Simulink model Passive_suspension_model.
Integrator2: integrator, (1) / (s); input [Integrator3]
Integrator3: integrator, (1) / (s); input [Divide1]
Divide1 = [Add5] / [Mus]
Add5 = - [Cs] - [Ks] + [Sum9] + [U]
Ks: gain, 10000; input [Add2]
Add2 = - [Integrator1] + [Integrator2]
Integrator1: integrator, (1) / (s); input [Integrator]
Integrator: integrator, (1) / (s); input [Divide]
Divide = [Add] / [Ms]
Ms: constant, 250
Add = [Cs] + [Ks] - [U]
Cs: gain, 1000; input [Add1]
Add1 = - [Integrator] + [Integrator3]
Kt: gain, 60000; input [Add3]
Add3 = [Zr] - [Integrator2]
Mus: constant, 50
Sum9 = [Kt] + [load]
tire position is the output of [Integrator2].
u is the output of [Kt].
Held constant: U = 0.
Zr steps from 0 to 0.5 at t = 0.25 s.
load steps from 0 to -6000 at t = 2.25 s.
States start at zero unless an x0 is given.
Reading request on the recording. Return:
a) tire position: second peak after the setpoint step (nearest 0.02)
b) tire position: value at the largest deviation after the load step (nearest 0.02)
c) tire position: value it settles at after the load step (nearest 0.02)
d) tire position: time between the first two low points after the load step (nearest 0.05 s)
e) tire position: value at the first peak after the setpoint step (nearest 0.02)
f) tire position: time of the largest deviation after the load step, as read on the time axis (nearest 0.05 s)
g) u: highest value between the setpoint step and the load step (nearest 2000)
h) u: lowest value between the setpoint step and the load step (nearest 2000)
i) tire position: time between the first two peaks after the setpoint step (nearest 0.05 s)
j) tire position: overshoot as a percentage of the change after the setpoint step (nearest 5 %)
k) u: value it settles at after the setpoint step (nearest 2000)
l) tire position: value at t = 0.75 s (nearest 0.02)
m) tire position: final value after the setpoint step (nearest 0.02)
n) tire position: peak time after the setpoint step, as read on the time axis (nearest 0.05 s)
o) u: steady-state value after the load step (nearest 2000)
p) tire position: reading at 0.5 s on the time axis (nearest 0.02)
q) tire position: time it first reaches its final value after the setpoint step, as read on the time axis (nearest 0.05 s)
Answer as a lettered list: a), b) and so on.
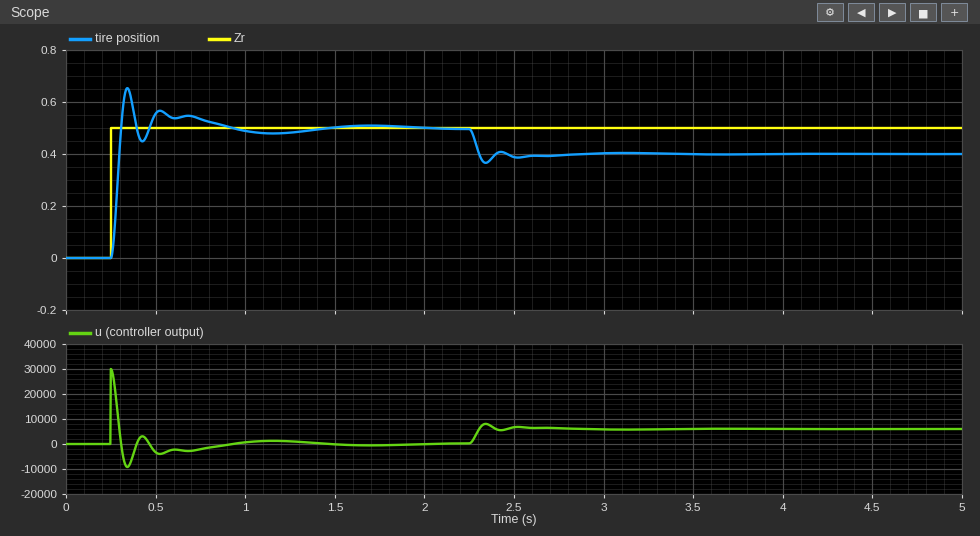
a) 0.56
b) 0.36
c) 0.40
d) 0.20 s
e) 0.66
f) 2.35 s
g) 30000
h) -10000
i) 0.20 s
j) 30 %
k) 0
l) 0.54
m) 0.50
n) 0.35 s
o) 6000
p) 0.56
q) 0.30 s
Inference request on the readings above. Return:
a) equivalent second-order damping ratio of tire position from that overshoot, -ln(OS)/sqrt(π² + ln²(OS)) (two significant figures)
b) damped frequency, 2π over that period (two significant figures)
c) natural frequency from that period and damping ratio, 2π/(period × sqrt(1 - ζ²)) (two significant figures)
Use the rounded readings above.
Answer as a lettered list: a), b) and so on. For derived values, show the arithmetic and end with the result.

a) ln(0.3) = -1.204; 1.204 / sqrt(9.870 + 1.450) = 0.36
b) 2π / 0.2 = 31 rad/s
c) 2π / (0.2 × sqrt(1 - 0.36²)) = 34 rad/s
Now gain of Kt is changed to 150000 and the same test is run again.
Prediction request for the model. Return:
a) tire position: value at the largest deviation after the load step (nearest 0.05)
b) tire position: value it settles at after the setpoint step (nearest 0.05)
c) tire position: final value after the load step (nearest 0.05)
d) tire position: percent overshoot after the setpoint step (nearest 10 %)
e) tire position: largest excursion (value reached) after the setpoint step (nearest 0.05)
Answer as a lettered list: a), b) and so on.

a) 0.45
b) 0.50
c) 0.45
d) 50 %
e) 0.75
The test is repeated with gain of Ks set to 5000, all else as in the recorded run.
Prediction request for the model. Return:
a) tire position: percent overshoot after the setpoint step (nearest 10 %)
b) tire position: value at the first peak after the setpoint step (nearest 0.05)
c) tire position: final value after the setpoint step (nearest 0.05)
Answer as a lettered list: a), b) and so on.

a) 40 %
b) 0.70
c) 0.50
